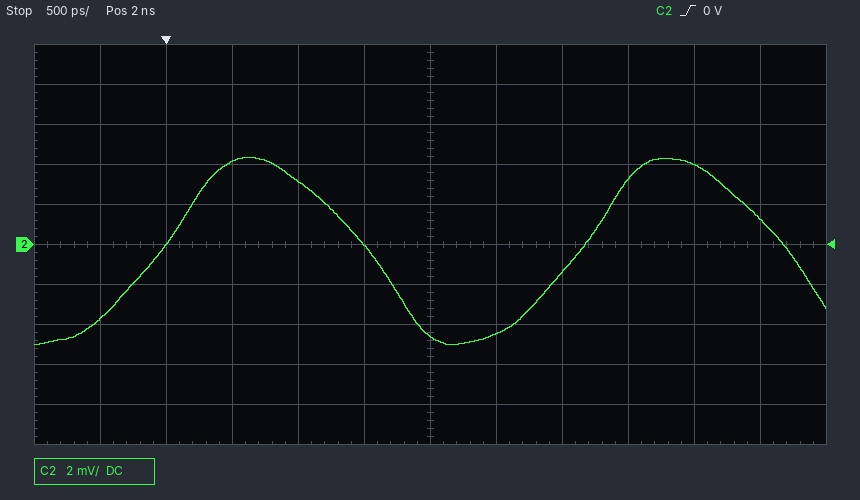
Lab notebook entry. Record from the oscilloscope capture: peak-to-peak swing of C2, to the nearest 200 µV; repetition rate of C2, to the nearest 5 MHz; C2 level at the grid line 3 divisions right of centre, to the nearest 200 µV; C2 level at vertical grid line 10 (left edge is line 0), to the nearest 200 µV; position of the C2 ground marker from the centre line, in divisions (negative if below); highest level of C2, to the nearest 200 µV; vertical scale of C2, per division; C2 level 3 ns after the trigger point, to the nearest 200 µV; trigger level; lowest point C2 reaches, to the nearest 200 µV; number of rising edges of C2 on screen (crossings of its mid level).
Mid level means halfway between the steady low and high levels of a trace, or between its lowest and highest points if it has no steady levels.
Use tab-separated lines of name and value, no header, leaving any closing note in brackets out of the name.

peak-to-peak swing of C2, to the nearest 200 µV	9.4 mV
repetition rate of C2, to the nearest 5 MHz	315 MHz
C2 level at the grid line 3 divisions right of centre, to the nearest 200 µV	3.2 mV
C2 level at vertical grid line 10 (left edge is line 0), to the nearest 200 µV	4.0 mV
position of the C2 ground marker from the centre line, in divisions	0.0 div
highest level of C2, to the nearest 200 µV	4.4 mV
vertical scale of C2, per division	2 mV
C2 level 3 ns after the trigger point, to the nearest 200 µV	-1.4 mV
trigger level	0 V
lowest point C2 reaches, to the nearest 200 µV	-5.0 mV
number of rising edges of C2 on screen	2
